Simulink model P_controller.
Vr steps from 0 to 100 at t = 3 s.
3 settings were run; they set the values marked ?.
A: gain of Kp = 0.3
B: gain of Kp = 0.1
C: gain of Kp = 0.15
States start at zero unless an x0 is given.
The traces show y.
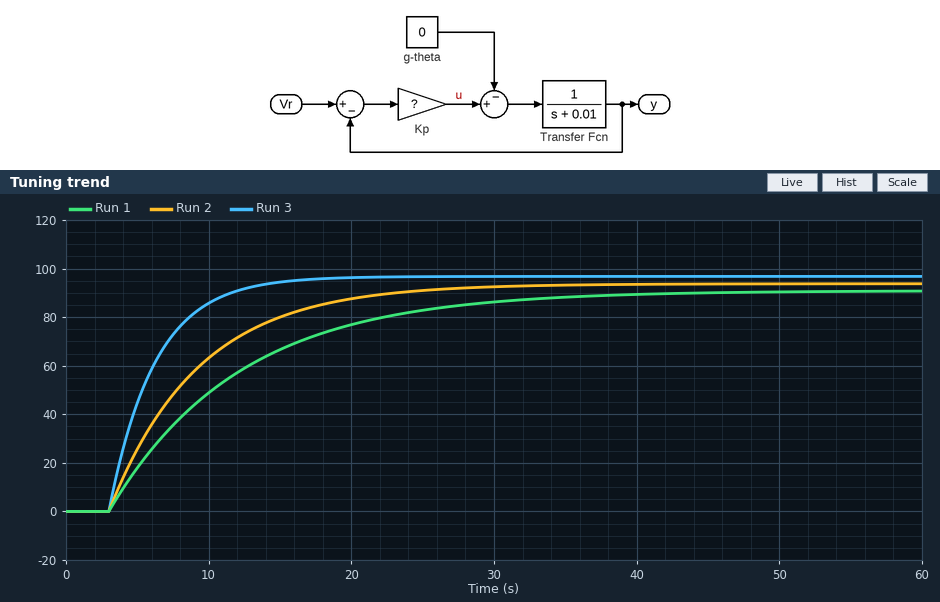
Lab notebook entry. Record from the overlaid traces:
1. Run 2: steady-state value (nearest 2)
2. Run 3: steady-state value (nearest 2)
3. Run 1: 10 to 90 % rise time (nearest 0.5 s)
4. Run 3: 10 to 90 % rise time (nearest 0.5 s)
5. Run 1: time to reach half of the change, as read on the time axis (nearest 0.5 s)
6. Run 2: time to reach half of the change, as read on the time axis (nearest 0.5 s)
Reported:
94
96
20.0 s
7.0 s
9.5 s
7.5 s
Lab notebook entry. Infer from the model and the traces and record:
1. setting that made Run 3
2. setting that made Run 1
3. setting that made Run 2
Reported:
A
B
C
